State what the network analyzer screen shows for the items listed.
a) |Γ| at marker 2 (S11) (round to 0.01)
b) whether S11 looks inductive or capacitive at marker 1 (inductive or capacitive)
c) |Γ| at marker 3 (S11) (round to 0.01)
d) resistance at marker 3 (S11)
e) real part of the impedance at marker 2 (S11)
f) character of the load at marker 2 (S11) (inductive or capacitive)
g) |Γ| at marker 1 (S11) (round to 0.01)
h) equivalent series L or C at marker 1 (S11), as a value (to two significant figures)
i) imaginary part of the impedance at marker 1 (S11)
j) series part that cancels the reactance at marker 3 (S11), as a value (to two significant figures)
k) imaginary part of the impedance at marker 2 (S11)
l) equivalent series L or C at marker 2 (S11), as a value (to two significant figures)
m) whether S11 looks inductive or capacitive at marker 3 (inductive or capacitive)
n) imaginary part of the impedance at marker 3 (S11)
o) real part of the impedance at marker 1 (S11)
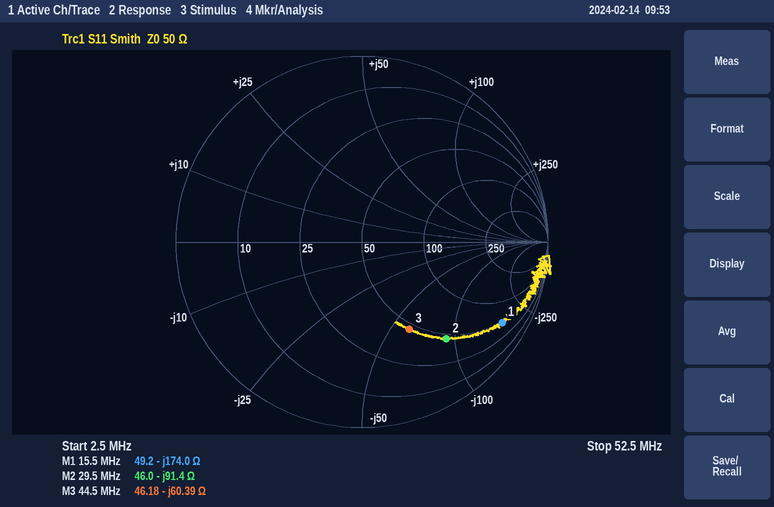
0.69
capacitive
0.53
46.18 Ω
46.0 Ω
capacitive
0.87
59 pF
-174.0 Ω
220 nH
-91.4 Ω
59 pF
capacitive
-60.39 Ω
49.2 Ω
